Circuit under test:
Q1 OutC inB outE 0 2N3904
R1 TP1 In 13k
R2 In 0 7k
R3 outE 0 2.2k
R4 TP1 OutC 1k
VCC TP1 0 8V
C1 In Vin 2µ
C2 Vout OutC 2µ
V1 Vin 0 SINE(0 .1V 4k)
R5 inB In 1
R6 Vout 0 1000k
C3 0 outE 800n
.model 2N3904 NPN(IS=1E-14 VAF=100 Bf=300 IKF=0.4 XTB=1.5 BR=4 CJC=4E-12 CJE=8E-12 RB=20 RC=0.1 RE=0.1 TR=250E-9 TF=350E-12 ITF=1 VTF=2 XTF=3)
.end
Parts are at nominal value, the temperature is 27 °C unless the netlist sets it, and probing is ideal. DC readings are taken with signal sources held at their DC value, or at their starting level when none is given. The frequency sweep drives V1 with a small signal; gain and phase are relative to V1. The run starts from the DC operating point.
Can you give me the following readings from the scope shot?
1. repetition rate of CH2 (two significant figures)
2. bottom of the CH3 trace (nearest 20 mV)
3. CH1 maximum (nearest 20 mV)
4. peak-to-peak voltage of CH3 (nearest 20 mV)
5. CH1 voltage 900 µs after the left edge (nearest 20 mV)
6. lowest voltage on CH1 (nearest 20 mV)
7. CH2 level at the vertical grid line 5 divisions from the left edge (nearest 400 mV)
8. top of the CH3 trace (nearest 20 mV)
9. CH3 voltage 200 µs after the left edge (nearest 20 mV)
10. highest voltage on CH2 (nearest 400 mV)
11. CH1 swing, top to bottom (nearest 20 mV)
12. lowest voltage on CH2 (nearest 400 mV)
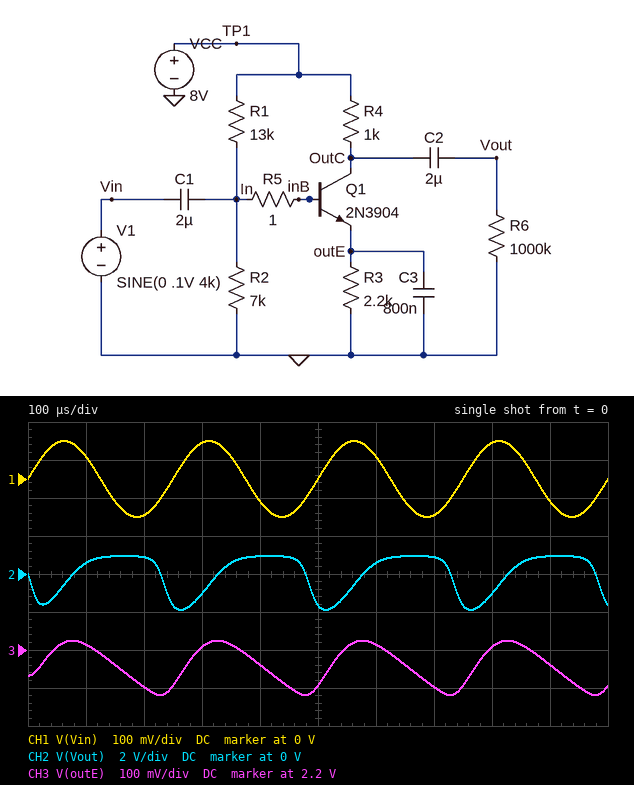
4.0 kHz
2.08 V
100 mV
140 mV
-60 mV
-100 mV
-1.6 V
2.22 V
2.10 V
800 mV
200 mV
-2.0 V
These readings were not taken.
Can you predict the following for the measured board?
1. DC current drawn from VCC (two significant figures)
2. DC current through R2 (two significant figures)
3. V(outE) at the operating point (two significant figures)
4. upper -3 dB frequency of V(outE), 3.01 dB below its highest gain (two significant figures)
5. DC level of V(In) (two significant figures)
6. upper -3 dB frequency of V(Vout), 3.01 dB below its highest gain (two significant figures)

1.4 mA
400 µA
2.1 V
7.5 kHz
2.8 V
39 MHz
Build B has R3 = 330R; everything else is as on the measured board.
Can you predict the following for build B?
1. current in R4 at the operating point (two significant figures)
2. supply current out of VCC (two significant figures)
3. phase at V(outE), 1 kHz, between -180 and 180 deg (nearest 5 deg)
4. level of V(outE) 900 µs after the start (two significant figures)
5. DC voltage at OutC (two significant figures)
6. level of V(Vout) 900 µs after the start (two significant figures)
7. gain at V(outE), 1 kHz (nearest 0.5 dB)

5.9 mA
6.3 mA
0 deg
1.8 V
2.1 V
2.2 V
-1.5 dB
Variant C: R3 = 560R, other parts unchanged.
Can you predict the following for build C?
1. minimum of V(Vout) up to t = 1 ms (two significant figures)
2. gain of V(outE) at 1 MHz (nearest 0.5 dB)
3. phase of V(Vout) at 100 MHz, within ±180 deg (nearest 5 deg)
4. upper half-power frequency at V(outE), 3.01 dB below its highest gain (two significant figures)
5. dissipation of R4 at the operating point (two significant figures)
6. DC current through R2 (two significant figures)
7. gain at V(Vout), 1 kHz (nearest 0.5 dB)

-2.0 V
-31.5 dB
85 deg
27 kHz
13 mW
390 µA
14.5 dB
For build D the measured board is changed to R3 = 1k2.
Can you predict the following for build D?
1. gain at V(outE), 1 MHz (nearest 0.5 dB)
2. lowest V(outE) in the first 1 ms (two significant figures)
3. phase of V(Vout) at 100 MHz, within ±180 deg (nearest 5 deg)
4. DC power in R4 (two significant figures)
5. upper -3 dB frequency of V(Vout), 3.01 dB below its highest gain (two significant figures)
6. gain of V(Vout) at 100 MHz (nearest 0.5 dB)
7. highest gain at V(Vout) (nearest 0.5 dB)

-37.5 dB
2.0 V
95 deg
3.1 mW
27 MHz
24.5 dB
36.5 dB
